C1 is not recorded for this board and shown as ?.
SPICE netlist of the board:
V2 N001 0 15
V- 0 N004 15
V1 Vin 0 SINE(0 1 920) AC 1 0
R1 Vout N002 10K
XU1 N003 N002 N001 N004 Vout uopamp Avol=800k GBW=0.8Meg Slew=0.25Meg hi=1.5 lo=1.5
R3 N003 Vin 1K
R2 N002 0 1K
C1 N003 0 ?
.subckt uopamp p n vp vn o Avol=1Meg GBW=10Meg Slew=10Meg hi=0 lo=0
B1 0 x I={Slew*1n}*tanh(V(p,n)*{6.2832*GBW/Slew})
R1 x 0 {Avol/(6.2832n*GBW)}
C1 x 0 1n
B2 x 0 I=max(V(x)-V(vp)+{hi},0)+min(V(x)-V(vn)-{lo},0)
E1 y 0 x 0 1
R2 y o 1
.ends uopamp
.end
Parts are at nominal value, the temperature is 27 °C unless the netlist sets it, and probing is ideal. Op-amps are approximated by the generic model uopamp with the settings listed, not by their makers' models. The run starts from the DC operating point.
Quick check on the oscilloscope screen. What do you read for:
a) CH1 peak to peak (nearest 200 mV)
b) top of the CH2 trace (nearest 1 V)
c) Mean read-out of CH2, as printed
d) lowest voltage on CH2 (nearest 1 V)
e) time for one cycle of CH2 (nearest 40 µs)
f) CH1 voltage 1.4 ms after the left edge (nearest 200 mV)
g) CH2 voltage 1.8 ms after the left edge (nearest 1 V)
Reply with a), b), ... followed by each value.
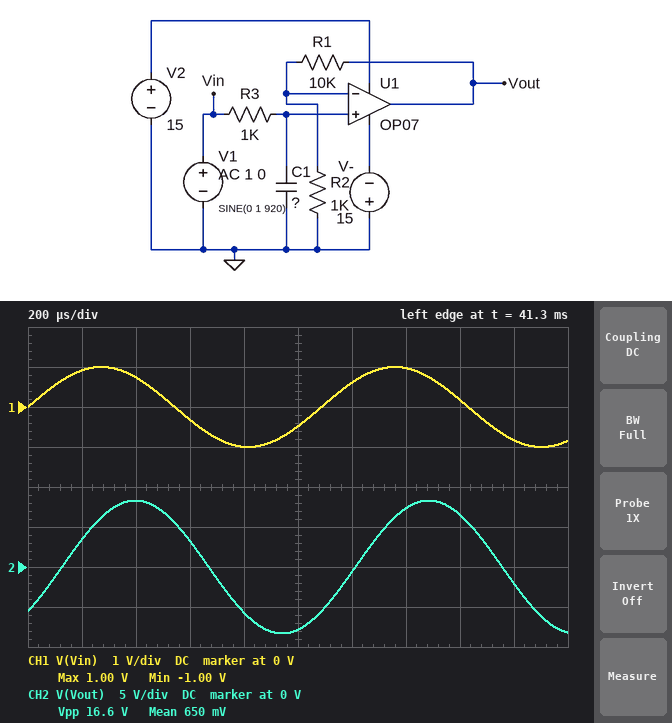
a) 2.0 V
b) 8 V
c) 650 mV
d) -8 V
e) 1.08 ms
f) 1.0 V
g) -2 V
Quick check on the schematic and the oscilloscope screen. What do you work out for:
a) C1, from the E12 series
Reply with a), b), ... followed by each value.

a) 150 nF
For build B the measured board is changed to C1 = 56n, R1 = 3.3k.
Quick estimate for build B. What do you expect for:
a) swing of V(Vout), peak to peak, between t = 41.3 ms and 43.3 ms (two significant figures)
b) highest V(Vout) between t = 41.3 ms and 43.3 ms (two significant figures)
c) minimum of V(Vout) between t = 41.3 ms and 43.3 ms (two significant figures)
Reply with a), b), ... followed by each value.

a) 8.2 V
b) 4.1 V
c) -4.1 V
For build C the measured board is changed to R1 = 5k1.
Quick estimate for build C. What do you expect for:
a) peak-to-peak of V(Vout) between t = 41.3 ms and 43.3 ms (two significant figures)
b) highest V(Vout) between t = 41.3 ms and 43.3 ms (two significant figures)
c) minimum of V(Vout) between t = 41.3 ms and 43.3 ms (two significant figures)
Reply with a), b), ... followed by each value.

a) 9.2 V
b) 4.6 V
c) -4.6 V
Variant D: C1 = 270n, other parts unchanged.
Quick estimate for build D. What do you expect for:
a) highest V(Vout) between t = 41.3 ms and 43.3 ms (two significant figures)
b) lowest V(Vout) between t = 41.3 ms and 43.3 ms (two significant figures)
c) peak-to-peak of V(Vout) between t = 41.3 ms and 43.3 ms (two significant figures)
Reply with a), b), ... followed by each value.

a) 5.9 V
b) -5.9 V
c) 12 V
